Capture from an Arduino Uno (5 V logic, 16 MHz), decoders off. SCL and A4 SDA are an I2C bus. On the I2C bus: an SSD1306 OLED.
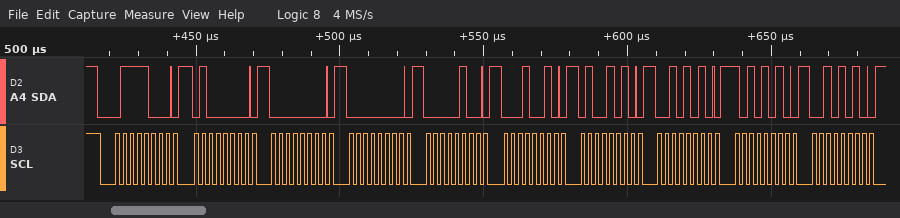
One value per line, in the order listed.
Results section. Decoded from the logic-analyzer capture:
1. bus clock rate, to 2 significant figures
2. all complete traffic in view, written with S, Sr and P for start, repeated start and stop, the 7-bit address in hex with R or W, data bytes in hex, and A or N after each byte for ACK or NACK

400 kHz
S 3CW A 40 A 00 A 00 A 04 A 12 A 4A A 2A A AA A 2A A
